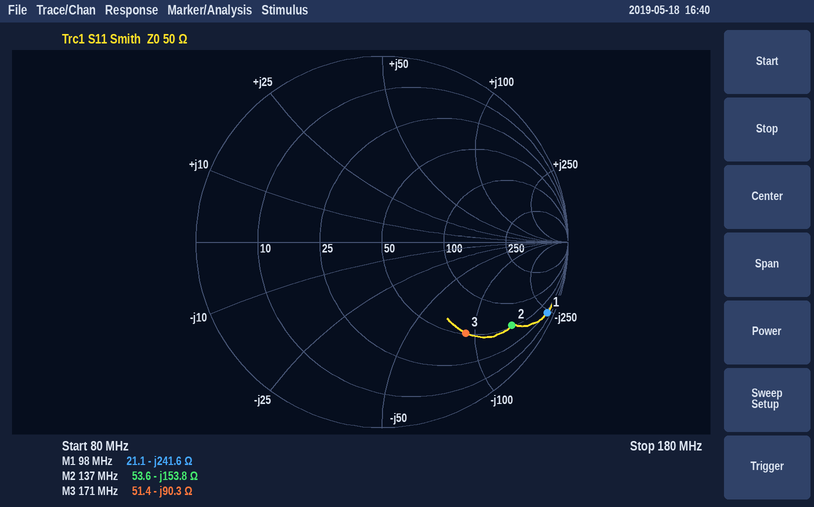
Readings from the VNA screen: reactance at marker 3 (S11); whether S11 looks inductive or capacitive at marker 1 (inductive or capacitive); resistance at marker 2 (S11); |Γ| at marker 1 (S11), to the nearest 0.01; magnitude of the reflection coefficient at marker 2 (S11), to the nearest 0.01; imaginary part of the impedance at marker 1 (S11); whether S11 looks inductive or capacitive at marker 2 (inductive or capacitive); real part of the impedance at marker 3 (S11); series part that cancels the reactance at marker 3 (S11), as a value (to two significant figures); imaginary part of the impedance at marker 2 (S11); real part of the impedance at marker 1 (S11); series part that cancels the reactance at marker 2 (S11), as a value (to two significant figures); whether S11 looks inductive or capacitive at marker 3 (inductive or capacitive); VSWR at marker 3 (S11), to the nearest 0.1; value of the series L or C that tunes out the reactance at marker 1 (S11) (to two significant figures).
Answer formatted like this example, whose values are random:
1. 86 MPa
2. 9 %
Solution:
1. -90.3 Ω
2. capacitive
3. 53.6 Ω
4. 0.97
5. 0.83
6. -241.6 Ω
7. capacitive
8. 51.4 Ω
9. 84 nH
10. -153.8 Ω
11. 21.1 Ω
12. 180 nH
13. capacitive
14. 5.0
15. 390 nH
